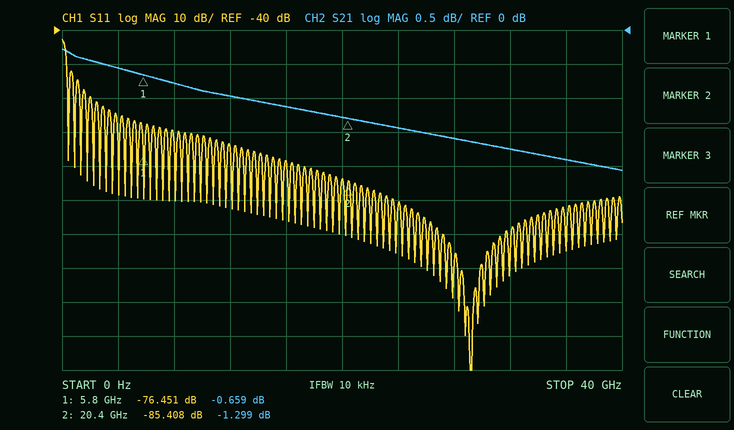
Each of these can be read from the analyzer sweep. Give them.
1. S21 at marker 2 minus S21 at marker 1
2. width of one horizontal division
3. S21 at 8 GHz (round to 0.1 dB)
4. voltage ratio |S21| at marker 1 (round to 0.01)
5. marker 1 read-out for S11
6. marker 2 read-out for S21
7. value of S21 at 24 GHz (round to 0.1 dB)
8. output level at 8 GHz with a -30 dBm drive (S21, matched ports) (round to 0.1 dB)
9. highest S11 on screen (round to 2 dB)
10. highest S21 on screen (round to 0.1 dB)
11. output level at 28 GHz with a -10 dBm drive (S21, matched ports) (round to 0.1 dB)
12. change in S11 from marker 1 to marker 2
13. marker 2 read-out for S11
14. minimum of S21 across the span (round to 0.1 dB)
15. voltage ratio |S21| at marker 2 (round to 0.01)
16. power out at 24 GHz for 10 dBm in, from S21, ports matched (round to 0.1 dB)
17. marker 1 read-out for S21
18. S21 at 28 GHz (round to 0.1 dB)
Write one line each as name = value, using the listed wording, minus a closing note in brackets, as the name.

S21 at marker 2 minus S21 at marker 1 = -0.640 dB
width of one horizontal division = 4 GHz
S21 at 8 GHz = -0.8 dB
voltage ratio |S21| at marker 1 = 0.93
marker 1 read-out for S11 = -76.451 dB
marker 2 read-out for S21 = -1.299 dB
value of S21 at 24 GHz = -1.4 dB
output level at 8 GHz with a -30 dBm drive (S21, matched ports) = -30.8 dBm
highest S11 on screen = -42 dB
highest S21 on screen = -0.3 dB
output level at 28 GHz with a -10 dBm drive (S21, matched ports) = -11.6 dBm
change in S11 from marker 1 to marker 2 = -8.957 dB
marker 2 read-out for S11 = -85.408 dB
minimum of S21 across the span = -2.1 dB
voltage ratio |S21| at marker 2 = 0.86
power out at 24 GHz for 10 dBm in, from S21, ports matched = 8.6 dBm
marker 1 read-out for S21 = -0.659 dB
S21 at 28 GHz = -1.6 dB
